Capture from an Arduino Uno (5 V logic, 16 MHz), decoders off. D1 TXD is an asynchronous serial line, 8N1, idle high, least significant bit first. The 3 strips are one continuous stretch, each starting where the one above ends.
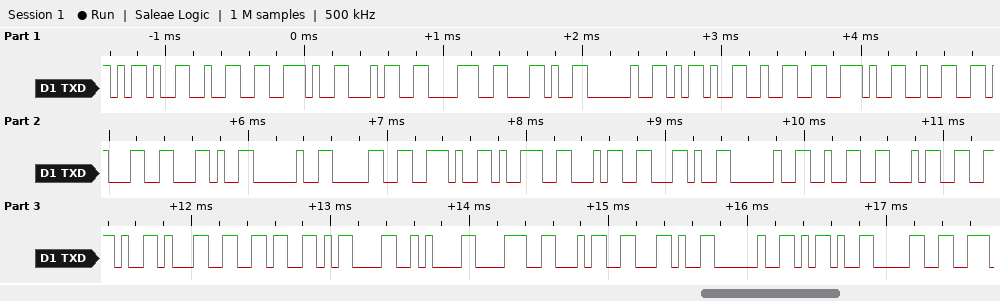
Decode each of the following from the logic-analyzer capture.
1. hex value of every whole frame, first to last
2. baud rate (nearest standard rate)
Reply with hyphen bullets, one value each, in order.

- 2D 32 2E 34 38 2C 20 2D 32 2E 32 31 2C 20 30 2E 39 34 2C 20 32 34 2E 31 36 0D 0A 38 34 2C 20 2D 30
- 19200 baud
